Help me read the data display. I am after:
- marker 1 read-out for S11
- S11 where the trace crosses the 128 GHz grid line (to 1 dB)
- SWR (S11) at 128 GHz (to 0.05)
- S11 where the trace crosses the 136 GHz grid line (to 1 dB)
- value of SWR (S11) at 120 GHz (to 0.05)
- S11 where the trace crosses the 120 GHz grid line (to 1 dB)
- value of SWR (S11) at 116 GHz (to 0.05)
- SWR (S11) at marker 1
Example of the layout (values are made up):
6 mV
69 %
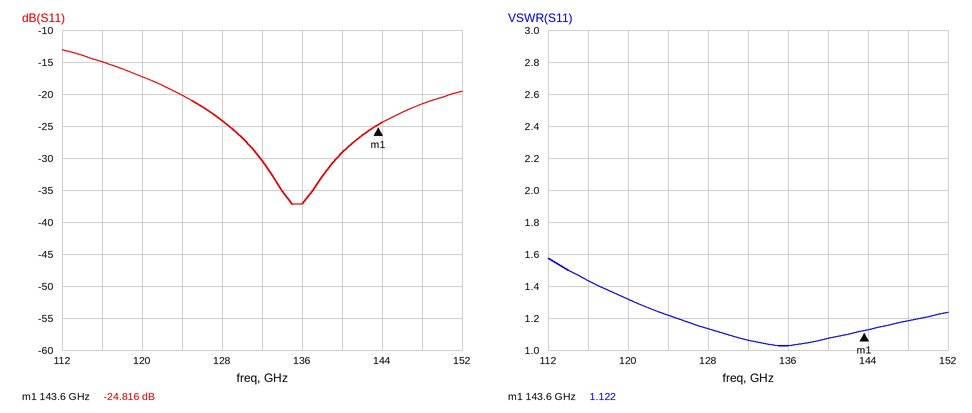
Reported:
-24.816 dB
-24 dB
1.15
-37 dB
1.30
-17 dB
1.45
1.122
